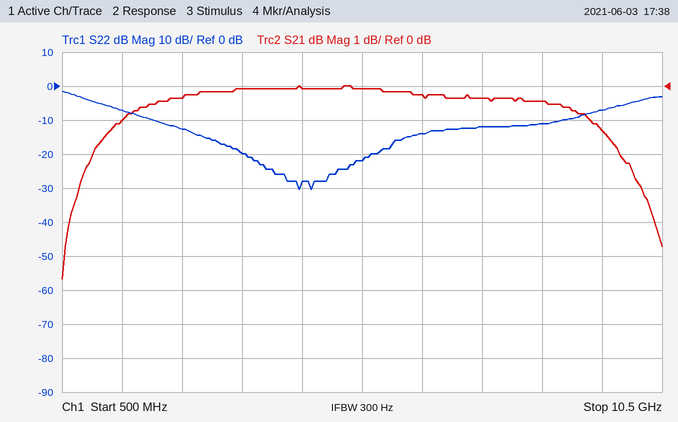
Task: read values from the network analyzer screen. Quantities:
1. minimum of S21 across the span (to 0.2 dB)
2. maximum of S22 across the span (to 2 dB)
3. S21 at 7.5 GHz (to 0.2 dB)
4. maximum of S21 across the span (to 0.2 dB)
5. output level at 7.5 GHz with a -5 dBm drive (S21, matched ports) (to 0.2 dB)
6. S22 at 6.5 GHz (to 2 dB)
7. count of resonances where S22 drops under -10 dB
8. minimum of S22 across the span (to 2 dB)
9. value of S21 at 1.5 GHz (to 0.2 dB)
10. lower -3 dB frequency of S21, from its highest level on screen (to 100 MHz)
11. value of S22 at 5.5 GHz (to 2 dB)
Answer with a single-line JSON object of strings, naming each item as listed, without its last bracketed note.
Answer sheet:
{"minimum of S21 across the span": "-5.6 dB", "maximum of S22 across the span": "-2 dB", "S21 at 7.5 GHz": "-0.4 dB", "maximum of S21 across the span": "0.0 dB", "output level at 7.5 GHz with a -5 dBm drive (S21, matched ports)": "-5.4 dBm", "S22 at 6.5 GHz": "-14 dB", "count of resonances where S22 drops under -10 dB": "2", "minimum of S22 across the span": "-30 dB", "value of S21 at 1.5 GHz": "-1.0 dB", "lower -3 dB frequency of S21, from its highest level on screen": "800 MHz", "value of S22 at 5.5 GHz": "-22 dB"}
